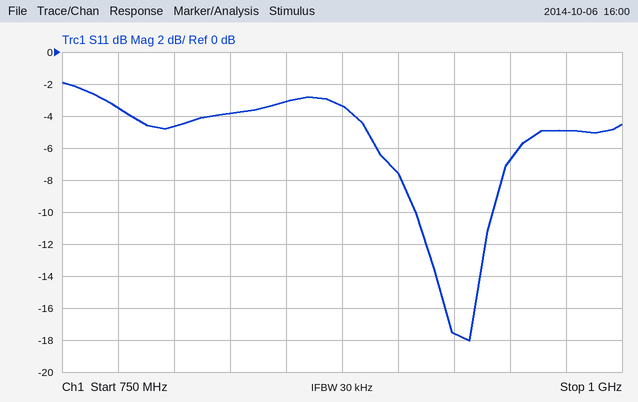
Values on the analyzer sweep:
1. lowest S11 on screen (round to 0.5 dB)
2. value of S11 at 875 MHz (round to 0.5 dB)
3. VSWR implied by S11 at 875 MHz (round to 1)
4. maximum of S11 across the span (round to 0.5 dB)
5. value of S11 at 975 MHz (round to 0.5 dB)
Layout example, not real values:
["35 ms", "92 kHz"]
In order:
["-18.0 dB", "-3.5 dB", "5", "-2.0 dB", "-5.0 dB"]
